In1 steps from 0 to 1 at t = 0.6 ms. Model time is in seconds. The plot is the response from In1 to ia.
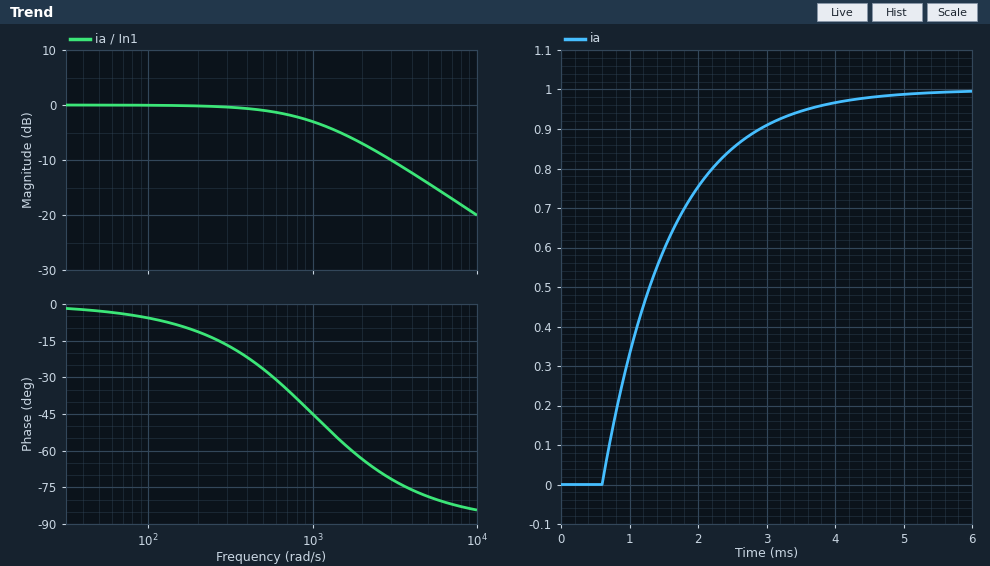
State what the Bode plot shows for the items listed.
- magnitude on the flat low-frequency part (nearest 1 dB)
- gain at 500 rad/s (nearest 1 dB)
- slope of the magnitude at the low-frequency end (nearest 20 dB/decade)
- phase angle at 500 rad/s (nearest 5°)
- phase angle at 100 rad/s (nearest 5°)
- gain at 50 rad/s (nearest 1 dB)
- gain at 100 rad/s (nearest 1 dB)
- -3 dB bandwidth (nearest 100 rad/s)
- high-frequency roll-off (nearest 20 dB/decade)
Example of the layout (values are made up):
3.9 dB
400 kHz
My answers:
0 dB
-1 dB
0 dB/decade
-25°
-5°
0 dB
0 dB
1000 rad/s
-20 dB/decade
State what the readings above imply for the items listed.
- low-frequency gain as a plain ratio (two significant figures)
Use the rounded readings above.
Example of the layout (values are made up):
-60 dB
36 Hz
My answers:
1.0
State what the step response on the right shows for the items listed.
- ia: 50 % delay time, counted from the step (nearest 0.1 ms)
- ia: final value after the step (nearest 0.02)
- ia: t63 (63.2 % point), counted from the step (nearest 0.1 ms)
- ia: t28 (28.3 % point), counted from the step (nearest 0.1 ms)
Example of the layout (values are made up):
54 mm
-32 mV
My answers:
0.7 ms
1.00
1.0 ms
0.3 ms
